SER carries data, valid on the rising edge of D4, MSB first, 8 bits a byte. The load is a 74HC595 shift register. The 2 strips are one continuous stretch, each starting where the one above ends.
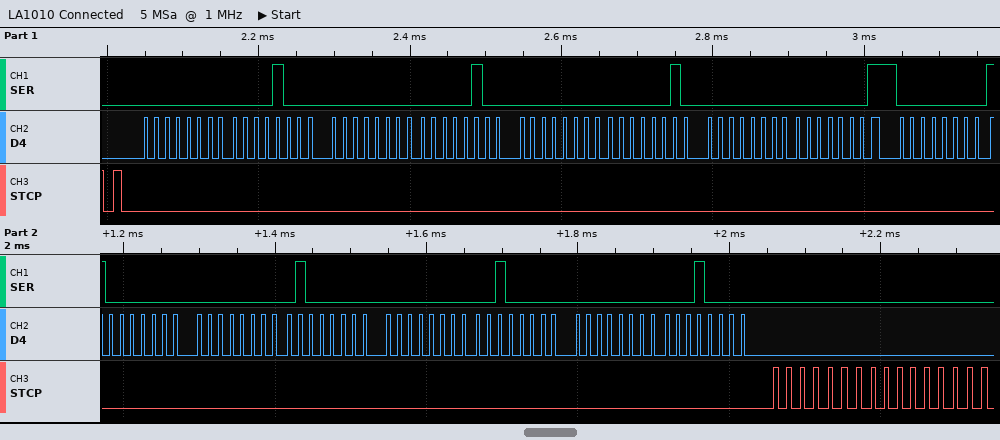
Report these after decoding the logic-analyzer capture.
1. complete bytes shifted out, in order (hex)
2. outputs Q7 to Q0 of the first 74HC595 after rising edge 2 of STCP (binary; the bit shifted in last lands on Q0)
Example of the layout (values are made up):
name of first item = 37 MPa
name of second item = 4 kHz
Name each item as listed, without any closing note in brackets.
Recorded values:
complete bytes shifted out, in order = 00 08 00 04 00 02 00 01 00 80 00 40 00 20 00 10
outputs Q7 to Q0 of the first 74HC595 after rising edge 2 of STCP = 00010000
